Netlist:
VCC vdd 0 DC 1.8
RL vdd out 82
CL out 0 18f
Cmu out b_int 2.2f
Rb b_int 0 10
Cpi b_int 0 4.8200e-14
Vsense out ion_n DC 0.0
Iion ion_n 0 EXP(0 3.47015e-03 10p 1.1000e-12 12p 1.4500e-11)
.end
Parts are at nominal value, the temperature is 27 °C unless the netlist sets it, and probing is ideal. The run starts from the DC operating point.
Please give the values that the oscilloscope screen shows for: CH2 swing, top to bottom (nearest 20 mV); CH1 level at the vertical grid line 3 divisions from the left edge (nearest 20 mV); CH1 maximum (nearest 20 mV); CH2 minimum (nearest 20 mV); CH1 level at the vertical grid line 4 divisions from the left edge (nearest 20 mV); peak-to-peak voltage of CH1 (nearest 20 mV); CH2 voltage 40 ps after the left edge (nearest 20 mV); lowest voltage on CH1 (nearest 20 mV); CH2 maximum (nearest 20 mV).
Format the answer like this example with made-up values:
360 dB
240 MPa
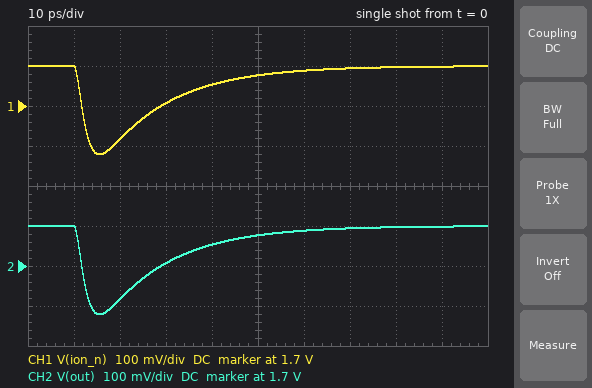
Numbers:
220 mV
1.70 V
1.80 V
1.58 V
1.76 V
220 mV
1.76 V
1.58 V
1.80 V
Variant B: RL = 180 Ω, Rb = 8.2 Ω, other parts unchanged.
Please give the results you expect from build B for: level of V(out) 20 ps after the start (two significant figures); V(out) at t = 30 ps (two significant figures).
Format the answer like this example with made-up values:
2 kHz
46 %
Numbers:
1.4 V
1.6 V
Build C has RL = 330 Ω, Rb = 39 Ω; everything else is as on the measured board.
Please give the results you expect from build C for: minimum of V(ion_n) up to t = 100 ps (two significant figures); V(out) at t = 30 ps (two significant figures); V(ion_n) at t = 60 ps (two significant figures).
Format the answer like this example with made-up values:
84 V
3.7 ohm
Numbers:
1.2 V
1.3 V
1.7 V
